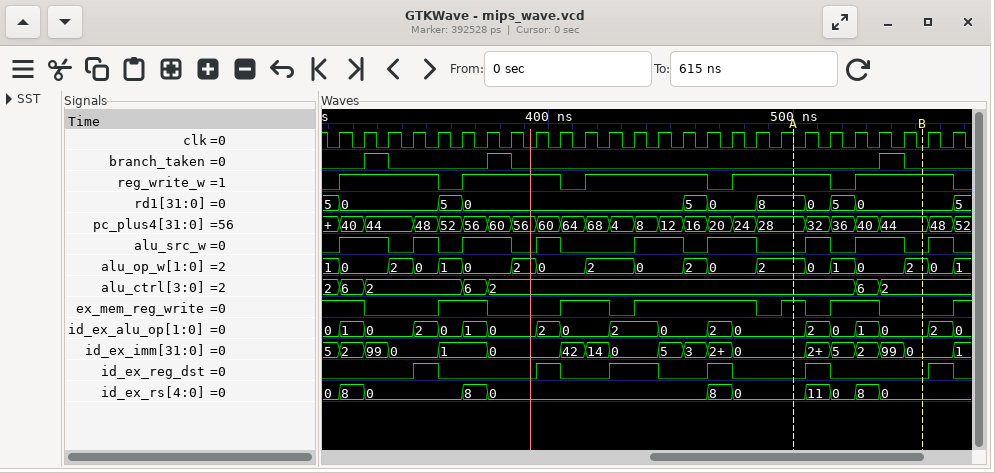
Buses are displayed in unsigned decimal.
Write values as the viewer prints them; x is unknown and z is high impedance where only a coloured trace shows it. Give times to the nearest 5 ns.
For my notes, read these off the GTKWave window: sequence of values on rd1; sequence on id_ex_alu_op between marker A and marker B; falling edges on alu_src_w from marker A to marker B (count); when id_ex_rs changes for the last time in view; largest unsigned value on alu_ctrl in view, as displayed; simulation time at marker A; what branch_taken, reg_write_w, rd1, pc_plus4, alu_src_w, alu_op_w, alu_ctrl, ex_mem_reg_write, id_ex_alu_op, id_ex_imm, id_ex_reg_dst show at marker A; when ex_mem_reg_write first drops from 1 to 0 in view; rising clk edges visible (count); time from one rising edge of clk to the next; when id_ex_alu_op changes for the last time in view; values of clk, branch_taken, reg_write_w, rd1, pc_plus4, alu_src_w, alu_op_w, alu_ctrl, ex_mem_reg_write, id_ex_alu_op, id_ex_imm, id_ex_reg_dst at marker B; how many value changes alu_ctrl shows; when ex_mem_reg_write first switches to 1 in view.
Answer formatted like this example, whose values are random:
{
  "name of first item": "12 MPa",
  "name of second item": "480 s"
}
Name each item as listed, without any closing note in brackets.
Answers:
{
  "sequence of values on rd1": "5, 0, 5, 0, 5, 0, 8, 0, 5, 0, 5",
  "sequence on id_ex_alu_op between marker A and marker B": "0, 2, 0, 1, 0",
  "falling edges on alu_src_w from marker A to marker B": "2",
  "when id_ex_rs changes for the last time in view": "535 ns",
  "largest unsigned value on alu_ctrl in view, as displayed": "6",
  "simulation time at marker A": "500 ns",
  "what branch_taken, reg_write_w, rd1, pc_plus4, alu_src_w, alu_op_w, alu_ctrl, ex_mem_reg_write, id_ex_alu_op, id_ex_imm, id_ex_reg_dst show at marker A": "branch_taken=0, reg_write_w=1, rd1=8, pc_plus4=28, alu_src_w=0, alu_op_w=2, alu_ctrl=2, ex_mem_reg_write=1, id_ex_alu_op=0, id_ex_imm=0, id_ex_reg_dst=0",
  "when ex_mem_reg_write first drops from 1 to 0 in view": "325 ns",
  "rising clk edges visible": "26",
  "time from one rising edge of clk to the next": "10 ns",
  "when id_ex_alu_op changes for the last time in view": "565 ns",
  "values of clk, branch_taken, reg_write_w, rd1, pc_plus4, alu_src_w, alu_op_w, alu_ctrl, ex_mem_reg_write, id_ex_alu_op, id_ex_imm, id_ex_reg_dst at marker B": "clk=0, branch_taken=0, reg_write_w=1, rd1=0, pc_plus4=44, alu_src_w=0, alu_op_w=2, alu_ctrl=2, ex_mem_reg_write=0, id_ex_alu_op=0, id_ex_imm=0, id_ex_reg_dst=0",
  "how many value changes alu_ctrl shows": "6",
  "when ex_mem_reg_write first switches to 1 in view": "355 ns"
}
